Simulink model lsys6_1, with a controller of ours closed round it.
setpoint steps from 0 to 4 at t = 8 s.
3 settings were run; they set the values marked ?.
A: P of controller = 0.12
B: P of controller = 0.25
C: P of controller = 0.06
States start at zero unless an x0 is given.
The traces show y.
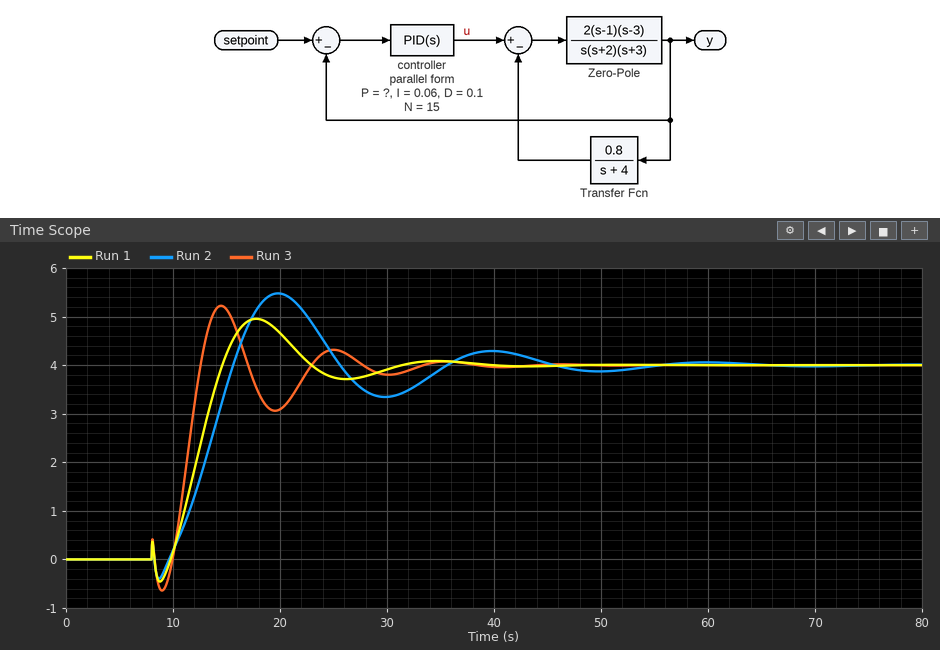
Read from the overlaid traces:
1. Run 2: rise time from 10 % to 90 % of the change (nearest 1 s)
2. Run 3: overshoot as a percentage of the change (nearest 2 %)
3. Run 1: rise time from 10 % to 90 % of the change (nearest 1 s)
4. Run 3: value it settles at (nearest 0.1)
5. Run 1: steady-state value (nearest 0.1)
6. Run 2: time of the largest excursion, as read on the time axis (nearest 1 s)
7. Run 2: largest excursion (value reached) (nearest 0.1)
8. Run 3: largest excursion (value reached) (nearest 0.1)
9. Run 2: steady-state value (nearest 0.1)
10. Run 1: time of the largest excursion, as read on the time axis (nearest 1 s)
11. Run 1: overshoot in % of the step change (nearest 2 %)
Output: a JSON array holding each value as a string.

["5 s", "30 %", "4 s", "4.0", "4.0", "20 s", "5.5", "5.2", "4.0", "18 s", "24 %"]
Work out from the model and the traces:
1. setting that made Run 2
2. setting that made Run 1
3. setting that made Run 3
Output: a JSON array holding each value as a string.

["C", "A", "B"]
